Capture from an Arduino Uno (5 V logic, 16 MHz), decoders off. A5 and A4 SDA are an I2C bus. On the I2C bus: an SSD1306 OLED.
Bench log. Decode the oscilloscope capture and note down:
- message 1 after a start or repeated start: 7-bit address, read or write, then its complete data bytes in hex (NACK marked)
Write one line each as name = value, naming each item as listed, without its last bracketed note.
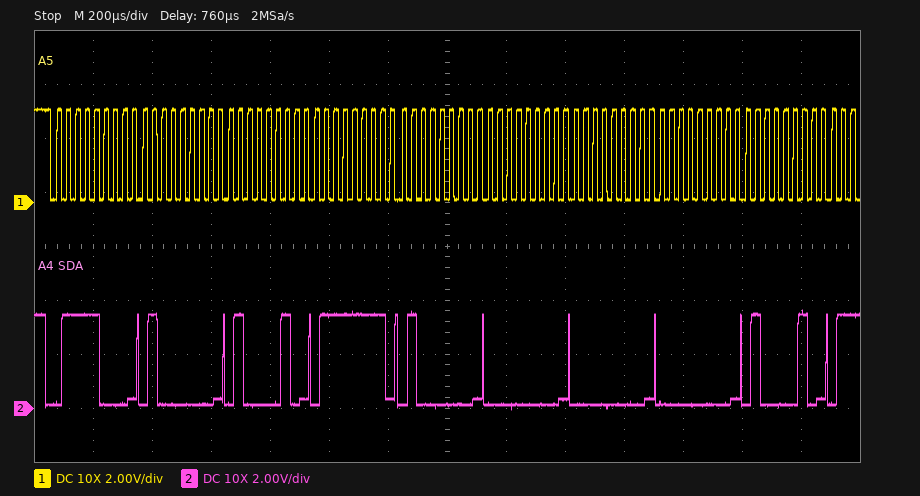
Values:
message 1 after a start or repeated start: 7-bit address, read or write, then its complete data bytes in hex = 0x3C write: 40 42 7F 40 00 00 00 42
